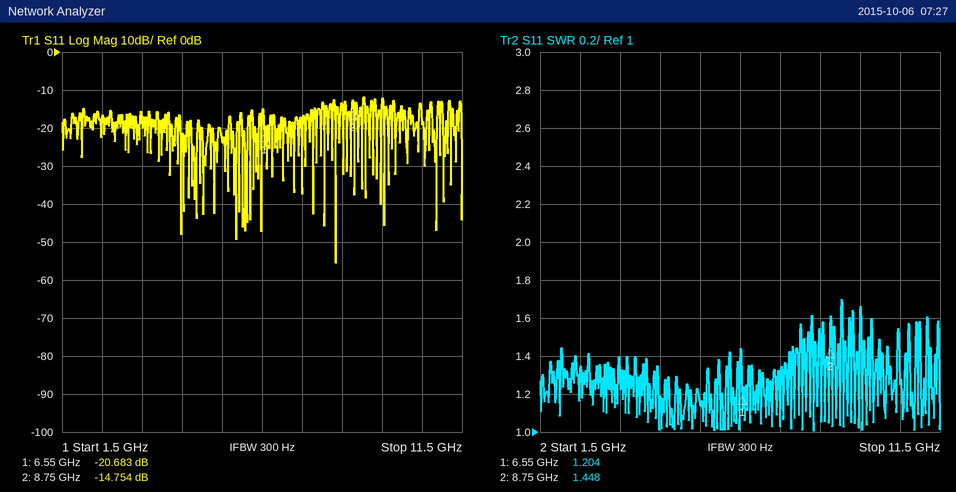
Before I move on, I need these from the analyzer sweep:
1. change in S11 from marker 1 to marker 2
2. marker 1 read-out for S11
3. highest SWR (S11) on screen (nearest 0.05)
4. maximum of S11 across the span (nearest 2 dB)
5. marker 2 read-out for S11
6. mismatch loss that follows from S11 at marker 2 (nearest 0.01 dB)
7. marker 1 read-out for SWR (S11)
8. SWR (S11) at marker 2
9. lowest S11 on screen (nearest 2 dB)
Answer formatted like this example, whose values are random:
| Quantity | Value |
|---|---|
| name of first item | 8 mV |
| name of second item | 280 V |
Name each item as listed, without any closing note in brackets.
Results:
| Quantity | Value |
|---|---|
| change in S11 from marker 1 to marker 2 | 5.929 dB |
| marker 1 read-out for S11 | -20.683 dB |
| highest SWR (S11) on screen | 1.70 |
| maximum of S11 across the span | -12 dB |
| marker 2 read-out for S11 | -14.754 dB |
| mismatch loss that follows from S11 at marker 2 | 0.15 dB |
| marker 1 read-out for SWR | 1.204 |
| SWR (S11) at marker 2 | 1.448 |
| lowest S11 on screen | -56 dB |
